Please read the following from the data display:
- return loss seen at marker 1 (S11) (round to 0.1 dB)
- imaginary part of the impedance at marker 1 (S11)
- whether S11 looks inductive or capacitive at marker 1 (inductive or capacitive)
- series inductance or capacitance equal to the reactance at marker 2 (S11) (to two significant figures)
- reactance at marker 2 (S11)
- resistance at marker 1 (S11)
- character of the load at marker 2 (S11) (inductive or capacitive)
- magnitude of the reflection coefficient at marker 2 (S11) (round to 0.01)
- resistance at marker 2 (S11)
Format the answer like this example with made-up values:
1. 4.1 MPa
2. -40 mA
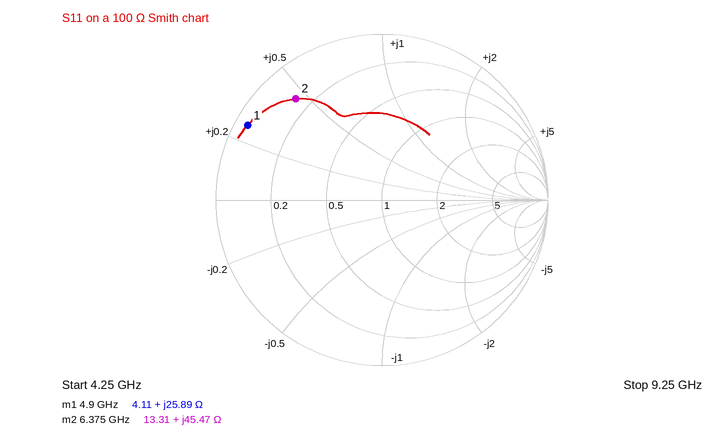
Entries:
1. 0.7 dB
2. +25.89 Ω
3. inductive
4. 1.1 nH
5. +45.47 Ω
6. 4.11 Ω
7. inductive
8. 0.80
9. 13.31 Ω
